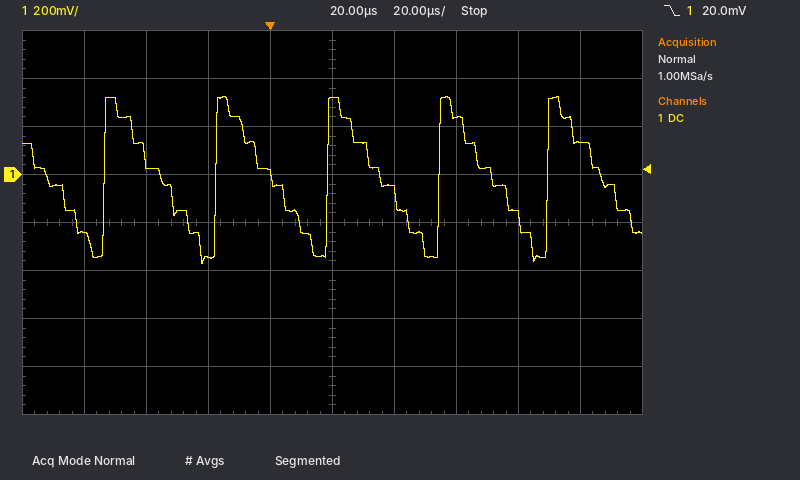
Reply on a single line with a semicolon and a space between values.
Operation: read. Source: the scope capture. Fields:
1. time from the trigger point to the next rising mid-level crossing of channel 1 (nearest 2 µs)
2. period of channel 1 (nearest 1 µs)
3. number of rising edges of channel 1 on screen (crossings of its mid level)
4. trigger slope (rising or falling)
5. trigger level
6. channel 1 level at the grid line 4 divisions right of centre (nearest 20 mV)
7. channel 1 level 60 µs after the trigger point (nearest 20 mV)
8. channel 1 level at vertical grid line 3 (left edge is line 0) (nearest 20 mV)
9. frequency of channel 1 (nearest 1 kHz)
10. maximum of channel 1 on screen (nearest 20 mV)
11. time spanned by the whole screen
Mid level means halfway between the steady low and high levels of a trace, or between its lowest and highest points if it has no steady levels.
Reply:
18 µs; 36 µs; 5; falling; 20.0 mV; 140 mV; 240 mV; -340 mV; 28 kHz; 320 mV; 200 µs
